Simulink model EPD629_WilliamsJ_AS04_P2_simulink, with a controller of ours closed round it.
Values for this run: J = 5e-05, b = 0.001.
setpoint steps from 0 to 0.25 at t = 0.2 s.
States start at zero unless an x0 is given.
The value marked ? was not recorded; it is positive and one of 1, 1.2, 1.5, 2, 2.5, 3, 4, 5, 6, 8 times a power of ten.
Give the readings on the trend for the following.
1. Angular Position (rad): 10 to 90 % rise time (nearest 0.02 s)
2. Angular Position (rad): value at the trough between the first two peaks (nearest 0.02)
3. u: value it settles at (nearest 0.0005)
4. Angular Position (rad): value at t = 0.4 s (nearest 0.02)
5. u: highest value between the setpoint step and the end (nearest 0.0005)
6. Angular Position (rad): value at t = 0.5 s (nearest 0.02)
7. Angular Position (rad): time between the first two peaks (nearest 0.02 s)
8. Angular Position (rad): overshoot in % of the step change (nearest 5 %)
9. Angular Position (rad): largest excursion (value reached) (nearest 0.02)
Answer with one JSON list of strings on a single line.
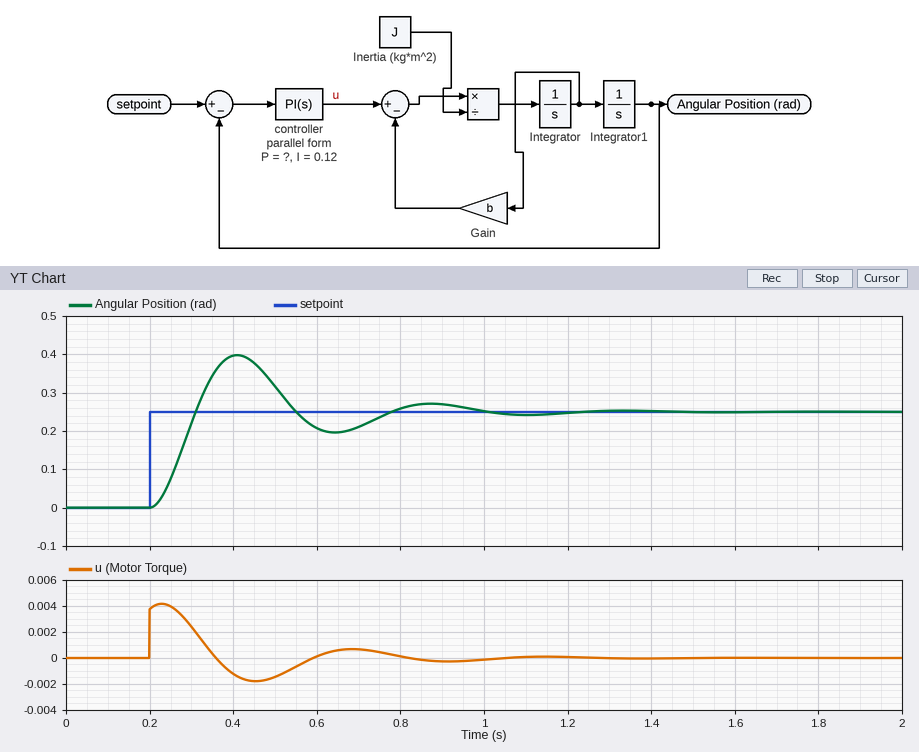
["0.08 s", "0.20", "0.0000", "0.40", "0.0040", "0.32", "0.46 s", "60 %", "0.40"]
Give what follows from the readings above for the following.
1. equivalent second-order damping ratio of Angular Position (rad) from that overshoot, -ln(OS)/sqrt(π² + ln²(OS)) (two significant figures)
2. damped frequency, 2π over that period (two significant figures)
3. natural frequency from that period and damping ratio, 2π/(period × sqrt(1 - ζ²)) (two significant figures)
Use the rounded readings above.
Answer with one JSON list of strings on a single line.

["0.16", "14 rad/s", "14 rad/s"]
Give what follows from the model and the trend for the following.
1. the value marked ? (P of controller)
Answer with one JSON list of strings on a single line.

["0.015"]
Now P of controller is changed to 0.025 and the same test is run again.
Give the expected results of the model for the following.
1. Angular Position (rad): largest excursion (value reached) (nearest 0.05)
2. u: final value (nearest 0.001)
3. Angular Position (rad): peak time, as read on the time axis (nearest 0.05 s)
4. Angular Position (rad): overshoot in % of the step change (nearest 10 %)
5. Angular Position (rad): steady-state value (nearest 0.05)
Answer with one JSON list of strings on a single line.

["0.35", "0.000", "0.35 s", "50 %", "0.25"]
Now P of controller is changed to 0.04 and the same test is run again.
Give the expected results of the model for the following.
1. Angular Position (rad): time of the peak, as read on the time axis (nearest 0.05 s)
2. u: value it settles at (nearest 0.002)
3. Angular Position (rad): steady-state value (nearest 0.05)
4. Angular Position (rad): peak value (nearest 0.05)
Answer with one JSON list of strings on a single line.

["0.30 s", "0.000", "0.25", "0.35"]
